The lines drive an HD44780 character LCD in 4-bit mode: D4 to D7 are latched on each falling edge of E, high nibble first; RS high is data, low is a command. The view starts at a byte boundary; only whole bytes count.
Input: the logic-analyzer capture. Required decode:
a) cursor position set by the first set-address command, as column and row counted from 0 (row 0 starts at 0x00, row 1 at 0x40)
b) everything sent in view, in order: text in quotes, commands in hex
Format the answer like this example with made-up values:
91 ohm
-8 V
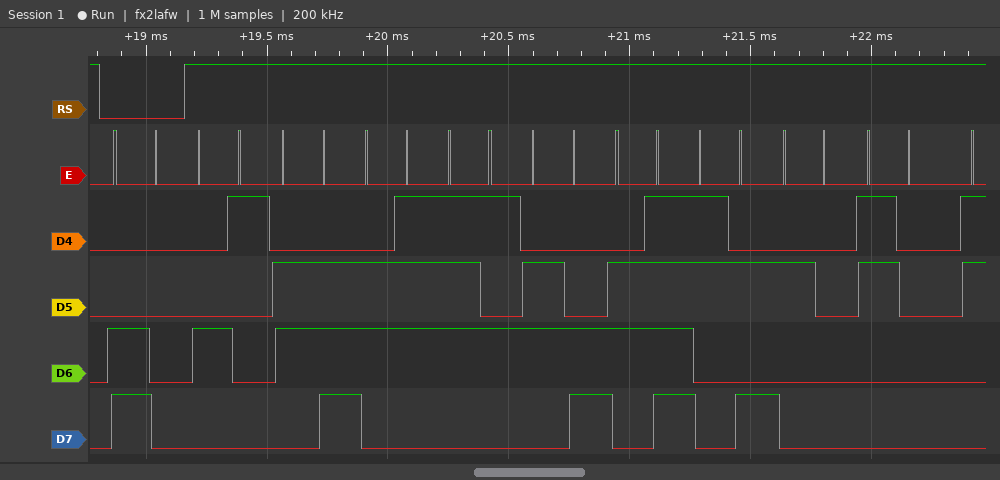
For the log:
column 0, row 1
0xC0 "Angulo: 0"
